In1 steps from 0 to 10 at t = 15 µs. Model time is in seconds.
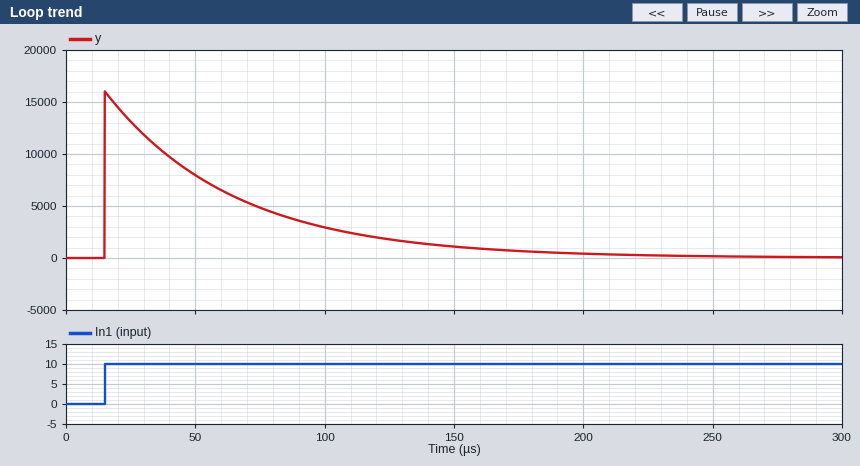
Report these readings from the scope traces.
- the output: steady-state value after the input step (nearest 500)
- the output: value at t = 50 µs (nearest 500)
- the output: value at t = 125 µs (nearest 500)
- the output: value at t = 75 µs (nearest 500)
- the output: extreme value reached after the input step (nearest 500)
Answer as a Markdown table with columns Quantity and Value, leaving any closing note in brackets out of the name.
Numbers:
| Quantity | Value |
|---|---|
| the output: steady-state value after the input step | 0 |
| the output: value at t = 50 µs | 8000 |
| the output: value at t = 125 µs | 2000 |
| the output: value at t = 75 µs | 5000 |
| the output: extreme value reached after the input step | 16000 |
